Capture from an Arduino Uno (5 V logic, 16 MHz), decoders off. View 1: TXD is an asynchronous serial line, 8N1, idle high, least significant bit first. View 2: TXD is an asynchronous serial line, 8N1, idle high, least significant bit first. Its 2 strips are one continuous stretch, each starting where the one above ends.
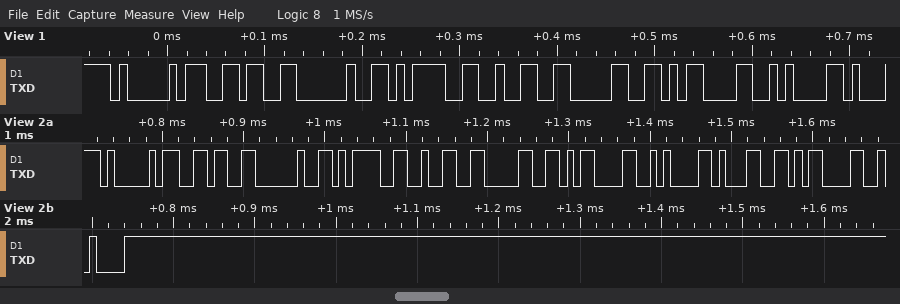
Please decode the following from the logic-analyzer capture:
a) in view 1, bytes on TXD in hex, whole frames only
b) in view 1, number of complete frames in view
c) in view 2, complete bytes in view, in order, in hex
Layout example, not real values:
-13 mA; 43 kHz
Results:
41 36 20 3D 32 30 0D 0A; 8; 0x41 0x36 0x20 0x3D 0x32 0x30 0x0D 0x0A 0x31 0x0D 0x0A
